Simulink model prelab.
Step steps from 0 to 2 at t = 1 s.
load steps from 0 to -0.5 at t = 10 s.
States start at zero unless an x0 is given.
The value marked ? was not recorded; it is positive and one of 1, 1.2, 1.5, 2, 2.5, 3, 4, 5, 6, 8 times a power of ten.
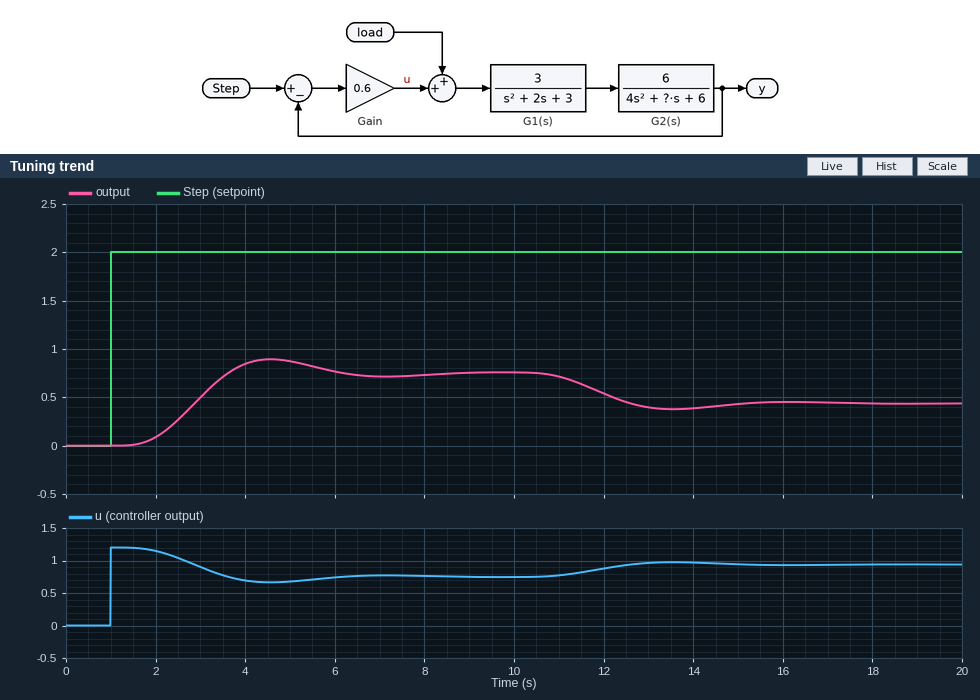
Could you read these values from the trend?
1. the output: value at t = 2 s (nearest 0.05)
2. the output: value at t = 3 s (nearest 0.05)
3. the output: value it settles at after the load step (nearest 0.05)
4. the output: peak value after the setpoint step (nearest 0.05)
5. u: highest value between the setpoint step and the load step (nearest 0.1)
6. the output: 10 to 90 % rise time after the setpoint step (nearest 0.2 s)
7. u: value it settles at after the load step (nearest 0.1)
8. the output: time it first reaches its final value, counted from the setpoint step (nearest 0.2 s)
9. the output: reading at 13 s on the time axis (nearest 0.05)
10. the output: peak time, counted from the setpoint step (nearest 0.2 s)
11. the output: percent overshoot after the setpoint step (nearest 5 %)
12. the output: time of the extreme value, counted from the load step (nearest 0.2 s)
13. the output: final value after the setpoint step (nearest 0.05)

0.10
0.50
0.45
0.90
1.2
1.4 s
0.9
2.6 s
0.40
3.6 s
20 %
3.6 s
0.75
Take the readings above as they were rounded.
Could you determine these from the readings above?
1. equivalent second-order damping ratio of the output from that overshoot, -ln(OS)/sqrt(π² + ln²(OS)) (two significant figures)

0.46
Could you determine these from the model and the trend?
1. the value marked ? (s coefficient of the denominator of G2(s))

10
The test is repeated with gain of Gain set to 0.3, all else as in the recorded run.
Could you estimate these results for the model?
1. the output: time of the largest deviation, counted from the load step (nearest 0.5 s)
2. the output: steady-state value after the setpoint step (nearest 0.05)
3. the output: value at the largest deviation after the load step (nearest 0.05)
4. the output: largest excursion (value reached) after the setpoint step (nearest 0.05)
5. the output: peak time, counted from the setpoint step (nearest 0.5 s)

4.0 s
0.45
0.05
0.50
4.0 s
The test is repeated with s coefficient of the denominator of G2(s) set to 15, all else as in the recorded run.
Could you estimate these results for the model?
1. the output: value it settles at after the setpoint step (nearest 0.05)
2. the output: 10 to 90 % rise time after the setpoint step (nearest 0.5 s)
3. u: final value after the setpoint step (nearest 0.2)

0.75
2.0 s
0.8
